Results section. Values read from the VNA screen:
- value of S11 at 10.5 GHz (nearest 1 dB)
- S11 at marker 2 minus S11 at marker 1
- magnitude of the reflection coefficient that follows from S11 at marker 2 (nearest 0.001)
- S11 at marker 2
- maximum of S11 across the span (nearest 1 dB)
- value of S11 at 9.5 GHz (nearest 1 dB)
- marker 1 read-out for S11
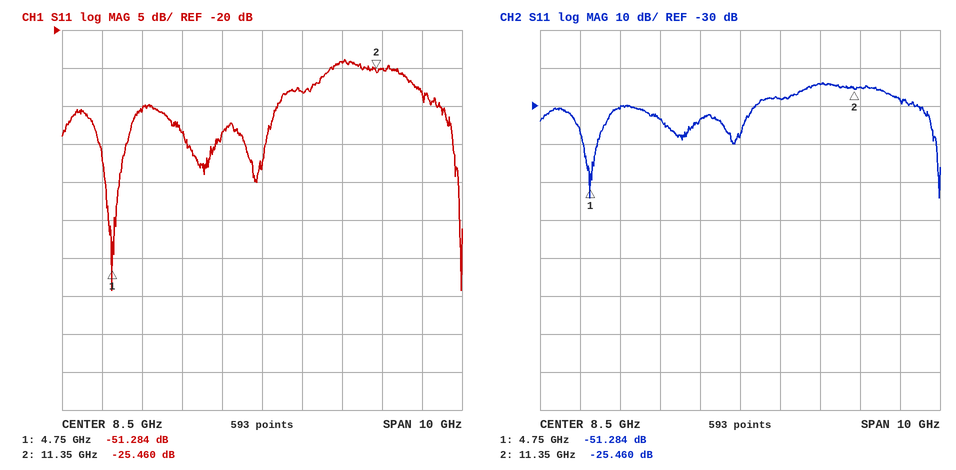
-24 dB
25.824 dB
0.053
-25.460 dB
-24 dB
-28 dB
-51.284 dB
